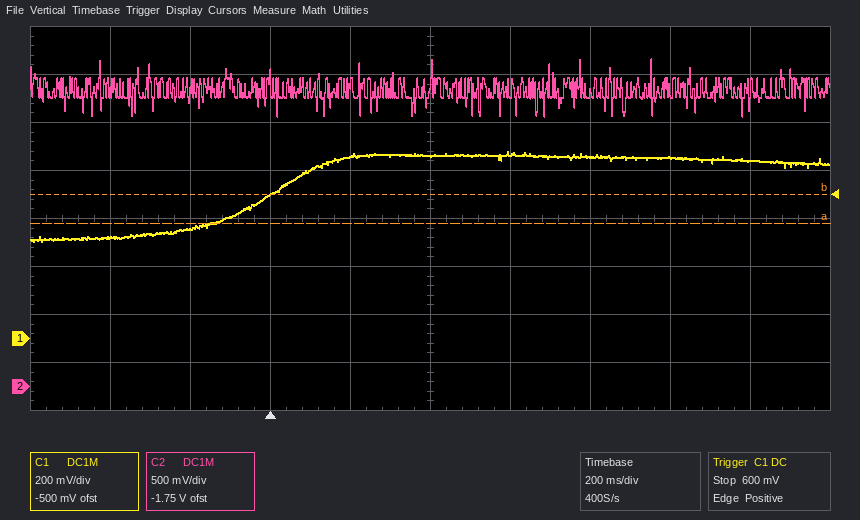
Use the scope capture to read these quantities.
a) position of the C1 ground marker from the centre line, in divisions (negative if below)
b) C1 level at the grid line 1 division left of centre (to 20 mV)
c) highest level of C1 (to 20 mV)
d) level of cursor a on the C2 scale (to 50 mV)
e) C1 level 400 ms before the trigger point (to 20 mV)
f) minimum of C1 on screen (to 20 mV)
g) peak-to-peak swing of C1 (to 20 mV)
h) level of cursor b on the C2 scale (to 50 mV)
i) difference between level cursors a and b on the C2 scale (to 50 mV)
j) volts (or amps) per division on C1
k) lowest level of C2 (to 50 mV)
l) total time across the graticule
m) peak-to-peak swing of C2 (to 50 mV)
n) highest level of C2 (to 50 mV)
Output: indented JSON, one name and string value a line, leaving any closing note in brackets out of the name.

{
  "position of the C1 ground marker from the centre line, in divisions": "-2.5 div",
  "C1 level at the grid line 1 division left of centre": "760 mV",
  "highest level of C1": "780 mV",
  "level of cursor a on the C2 scale": "1.70 V",
  "C1 level 400 ms before the trigger point": "420 mV",
  "minimum of C1 on screen": "400 mV",
  "peak-to-peak swing of C1": "380 mV",
  "level of cursor b on the C2 scale": "2.00 V",
  "difference between level cursors a and b on the C2 scale": "300 mV",
  "volts (or amps) per division on C1": "200 mV",
  "lowest level of C2": "2.80 V",
  "total time across the graticule": "2 s",
  "peak-to-peak swing of C2": "600 mV",
  "highest level of C2": "3.40 V"
}
